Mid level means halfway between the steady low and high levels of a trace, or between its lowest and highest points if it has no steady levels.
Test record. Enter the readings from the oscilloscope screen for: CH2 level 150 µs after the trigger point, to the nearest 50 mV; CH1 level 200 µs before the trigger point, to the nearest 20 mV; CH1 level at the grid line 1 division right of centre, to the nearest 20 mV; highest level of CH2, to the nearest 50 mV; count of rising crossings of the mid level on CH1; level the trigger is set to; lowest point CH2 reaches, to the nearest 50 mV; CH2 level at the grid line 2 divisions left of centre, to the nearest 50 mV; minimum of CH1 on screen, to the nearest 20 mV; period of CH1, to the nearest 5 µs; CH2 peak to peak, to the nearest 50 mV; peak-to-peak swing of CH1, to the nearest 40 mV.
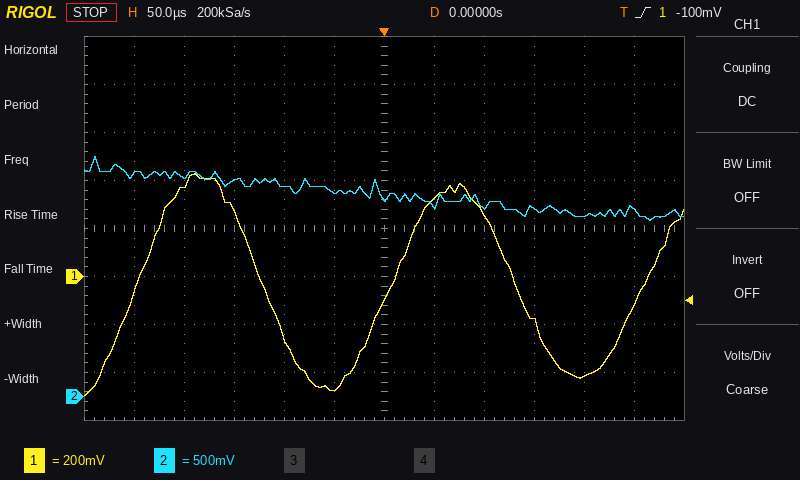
1.95 V
380 mV
320 mV
2.50 V
3
-100 mV
1.85 V
2.20 V
-500 mV
255 µs
650 mV
920 mV
